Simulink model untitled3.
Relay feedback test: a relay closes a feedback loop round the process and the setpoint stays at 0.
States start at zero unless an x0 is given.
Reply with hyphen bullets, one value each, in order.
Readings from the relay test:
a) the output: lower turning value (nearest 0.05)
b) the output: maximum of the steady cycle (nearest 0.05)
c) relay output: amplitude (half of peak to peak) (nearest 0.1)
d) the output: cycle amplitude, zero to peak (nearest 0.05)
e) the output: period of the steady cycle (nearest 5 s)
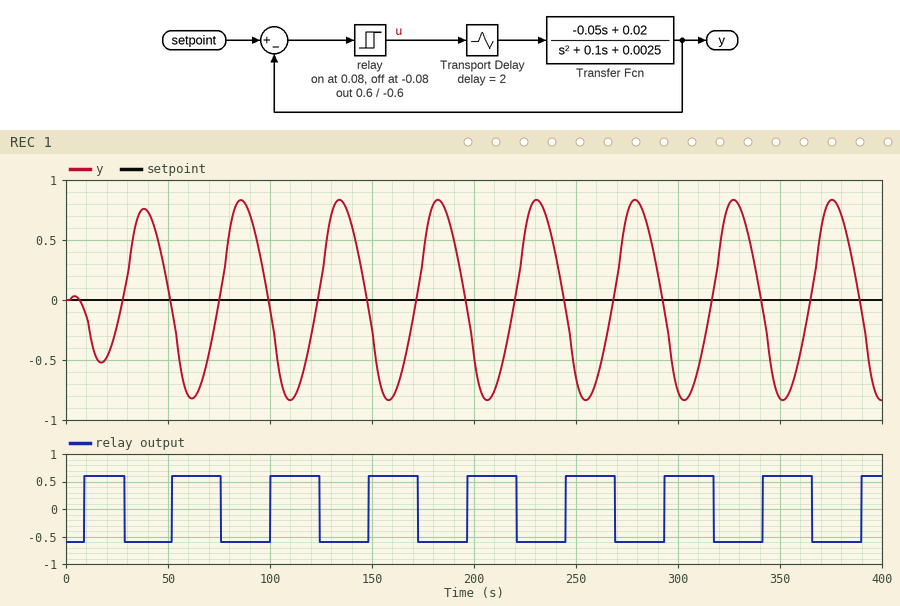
- -0.85
- 0.85
- 0.6
- 0.85
- 50 s
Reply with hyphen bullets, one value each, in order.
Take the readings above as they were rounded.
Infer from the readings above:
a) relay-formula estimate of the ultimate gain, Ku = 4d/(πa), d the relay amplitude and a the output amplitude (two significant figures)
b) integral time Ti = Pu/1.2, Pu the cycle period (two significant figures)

- 0.90
- 42 s
